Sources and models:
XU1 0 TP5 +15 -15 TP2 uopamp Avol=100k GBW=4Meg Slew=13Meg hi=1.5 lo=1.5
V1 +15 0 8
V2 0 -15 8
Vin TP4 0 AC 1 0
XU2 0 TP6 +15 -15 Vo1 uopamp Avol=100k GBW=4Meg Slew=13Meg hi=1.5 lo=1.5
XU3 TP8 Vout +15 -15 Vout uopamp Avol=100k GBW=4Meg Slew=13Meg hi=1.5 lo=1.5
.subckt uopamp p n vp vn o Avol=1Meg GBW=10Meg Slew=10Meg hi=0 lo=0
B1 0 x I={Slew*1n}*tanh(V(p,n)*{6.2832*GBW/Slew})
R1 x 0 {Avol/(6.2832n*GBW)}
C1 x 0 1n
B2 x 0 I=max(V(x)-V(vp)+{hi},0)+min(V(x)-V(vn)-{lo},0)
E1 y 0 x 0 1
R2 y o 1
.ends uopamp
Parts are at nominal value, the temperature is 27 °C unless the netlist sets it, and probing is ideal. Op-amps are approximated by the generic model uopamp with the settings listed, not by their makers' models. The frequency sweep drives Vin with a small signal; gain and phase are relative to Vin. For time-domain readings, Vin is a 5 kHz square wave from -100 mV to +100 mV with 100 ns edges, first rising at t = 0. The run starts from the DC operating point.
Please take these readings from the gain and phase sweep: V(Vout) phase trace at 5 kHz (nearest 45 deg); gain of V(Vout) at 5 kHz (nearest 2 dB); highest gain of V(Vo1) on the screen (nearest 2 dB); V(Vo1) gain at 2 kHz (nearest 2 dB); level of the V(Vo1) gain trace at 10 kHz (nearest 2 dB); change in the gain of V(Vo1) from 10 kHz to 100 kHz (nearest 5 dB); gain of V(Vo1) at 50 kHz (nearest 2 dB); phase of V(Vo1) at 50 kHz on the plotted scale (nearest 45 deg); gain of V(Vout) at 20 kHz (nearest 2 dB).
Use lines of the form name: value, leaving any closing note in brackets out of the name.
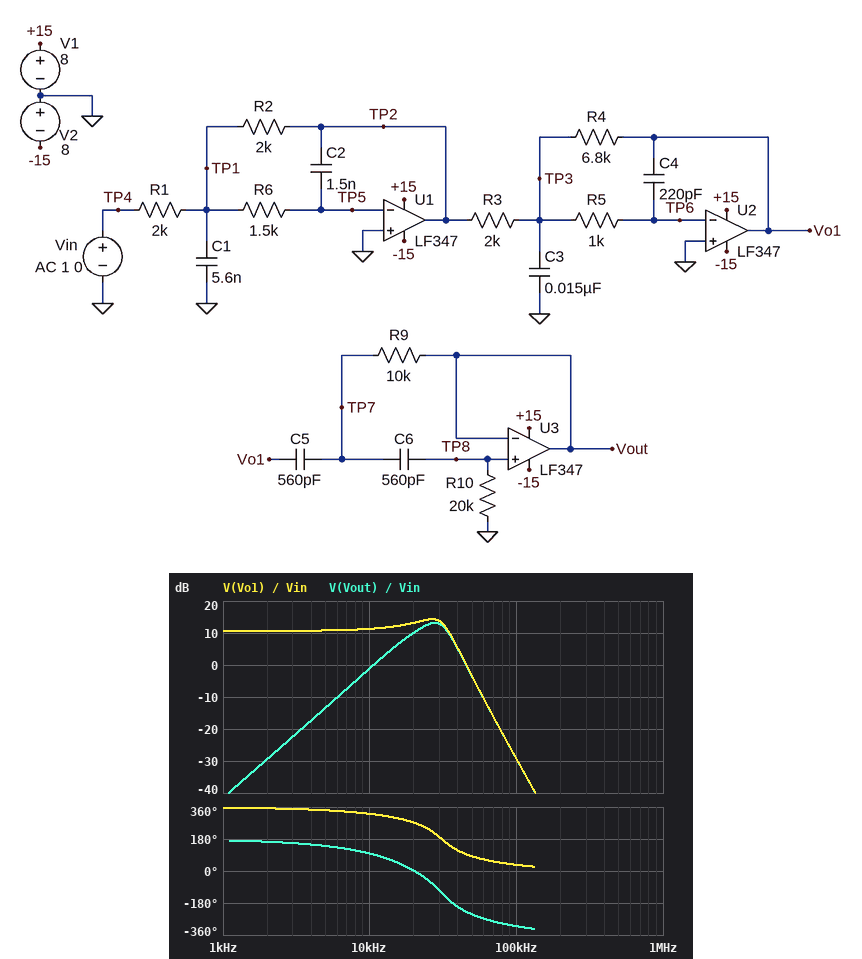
V(Vout) phase trace at 5 kHz: 135 deg
gain of V(Vout) at 5 kHz: -14 dB
highest gain of V(Vo1) on the screen: 14 dB
V(Vo1) gain at 2 kHz: 10 dB
level of the V(Vo1) gain trace at 10 kHz: 12 dB
change in the gain of V(Vo1) from 10 kHz to 100 kHz: -40 dB
gain of V(Vo1) at 50 kHz: -4 dB
phase of V(Vo1) at 50 kHz on the plotted scale: 90 deg
gain of V(Vout) at 20 kHz: 10 dB
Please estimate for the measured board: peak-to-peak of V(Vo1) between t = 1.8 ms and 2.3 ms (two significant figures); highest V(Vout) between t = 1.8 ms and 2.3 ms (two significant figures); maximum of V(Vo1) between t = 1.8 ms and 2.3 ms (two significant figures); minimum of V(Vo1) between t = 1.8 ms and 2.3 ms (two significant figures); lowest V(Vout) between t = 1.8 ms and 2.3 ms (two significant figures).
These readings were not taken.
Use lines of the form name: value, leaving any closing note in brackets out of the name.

peak-to-peak of V(Vo1) between t = 1.8 ms and 2.3 ms: 1.1 V
highest V(Vout) between t = 1.8 ms and 2.3 ms: 250 mV
maximum of V(Vo1) between t = 1.8 ms and 2.3 ms: 550 mV
minimum of V(Vo1) between t = 1.8 ms and 2.3 ms: -550 mV
lowest V(Vout) between t = 1.8 ms and 2.3 ms: -250 mV
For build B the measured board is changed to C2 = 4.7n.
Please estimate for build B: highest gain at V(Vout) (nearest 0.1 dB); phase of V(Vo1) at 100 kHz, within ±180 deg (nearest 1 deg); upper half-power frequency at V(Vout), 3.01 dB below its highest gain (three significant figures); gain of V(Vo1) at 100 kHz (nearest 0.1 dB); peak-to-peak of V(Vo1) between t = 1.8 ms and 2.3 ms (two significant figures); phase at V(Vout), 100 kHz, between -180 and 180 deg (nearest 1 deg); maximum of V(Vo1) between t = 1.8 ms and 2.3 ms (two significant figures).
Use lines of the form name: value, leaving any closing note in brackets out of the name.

highest gain at V(Vout): 3.0 dB
phase of V(Vo1) at 100 kHz, within ±180 deg: 33 deg
upper half-power frequency at V(Vout), 3.01 dB below its highest gain: 33.5 kHz
gain of V(Vo1) at 100 kHz: -39.6 dB
peak-to-peak of V(Vo1) between t = 1.8 ms and 2.3 ms: 670 mV
phase at V(Vout), 100 kHz, between -180 and 180 deg: 48 deg
maximum of V(Vo1) between t = 1.8 ms and 2.3 ms: 340 mV
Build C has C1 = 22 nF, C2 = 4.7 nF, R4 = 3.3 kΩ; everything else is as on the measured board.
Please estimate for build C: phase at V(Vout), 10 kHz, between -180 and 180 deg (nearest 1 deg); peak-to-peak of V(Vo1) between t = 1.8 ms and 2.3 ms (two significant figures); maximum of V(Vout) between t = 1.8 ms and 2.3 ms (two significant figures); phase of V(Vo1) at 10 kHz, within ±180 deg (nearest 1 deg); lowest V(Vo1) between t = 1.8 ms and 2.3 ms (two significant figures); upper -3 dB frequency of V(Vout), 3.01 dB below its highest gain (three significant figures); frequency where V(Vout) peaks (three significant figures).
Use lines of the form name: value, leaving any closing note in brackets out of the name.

phase at V(Vout), 10 kHz, between -180 and 180 deg: 32 deg
peak-to-peak of V(Vo1) between t = 1.8 ms and 2.3 ms: 370 mV
maximum of V(Vout) between t = 1.8 ms and 2.3 ms: 34 mV
phase of V(Vo1) at 10 kHz, within ±180 deg: -104 deg
lowest V(Vo1) between t = 1.8 ms and 2.3 ms: -190 mV
upper -3 dB frequency of V(Vout), 3.01 dB below its highest gain: 30.6 kHz
frequency where V(Vout) peaks: 14.4 kHz
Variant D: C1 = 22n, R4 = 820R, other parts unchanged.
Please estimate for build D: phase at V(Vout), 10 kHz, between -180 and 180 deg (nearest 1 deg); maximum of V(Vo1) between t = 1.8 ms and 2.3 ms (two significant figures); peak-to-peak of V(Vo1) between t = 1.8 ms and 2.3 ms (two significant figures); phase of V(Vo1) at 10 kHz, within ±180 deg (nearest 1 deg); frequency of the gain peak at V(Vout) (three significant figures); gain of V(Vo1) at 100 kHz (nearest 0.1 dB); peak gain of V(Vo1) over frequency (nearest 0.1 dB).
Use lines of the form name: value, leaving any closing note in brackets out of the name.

phase at V(Vout), 10 kHz, between -180 and 180 deg: 96 deg
maximum of V(Vo1) between t = 1.8 ms and 2.3 ms: 65 mV
peak-to-peak of V(Vo1) between t = 1.8 ms and 2.3 ms: 130 mV
phase of V(Vo1) at 10 kHz, within ±180 deg: -40 deg
frequency of the gain peak at V(Vout): 16.8 kHz
gain of V(Vo1) at 100 kHz: -32.0 dB
peak gain of V(Vo1) over frequency: -4.4 dB
